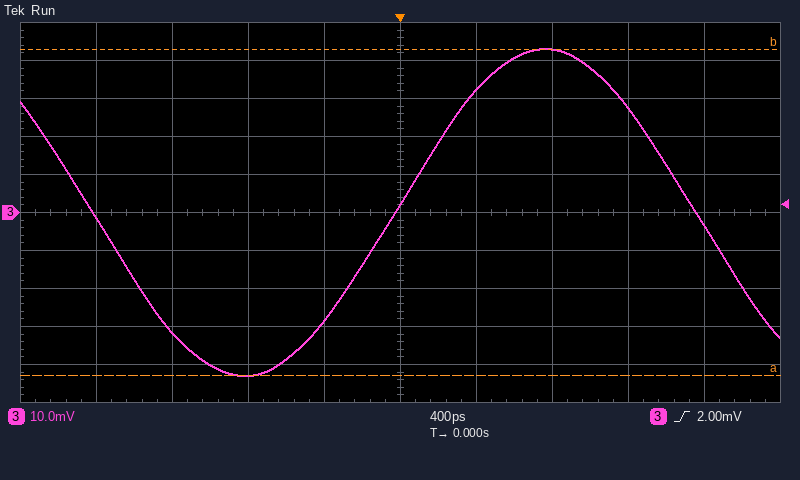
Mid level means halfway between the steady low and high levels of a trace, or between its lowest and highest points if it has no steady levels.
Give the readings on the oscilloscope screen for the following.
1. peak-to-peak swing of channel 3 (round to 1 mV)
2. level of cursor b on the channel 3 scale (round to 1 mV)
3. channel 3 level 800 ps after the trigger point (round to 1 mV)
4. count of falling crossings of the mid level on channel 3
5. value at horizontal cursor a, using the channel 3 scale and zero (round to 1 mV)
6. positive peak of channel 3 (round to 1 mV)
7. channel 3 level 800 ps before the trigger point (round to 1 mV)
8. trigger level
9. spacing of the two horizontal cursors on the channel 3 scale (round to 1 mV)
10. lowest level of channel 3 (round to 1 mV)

86 mV
43 mV
43 mV
2
-43 mV
43 mV
-43 mV
2.00 mV
86 mV
-43 mV
